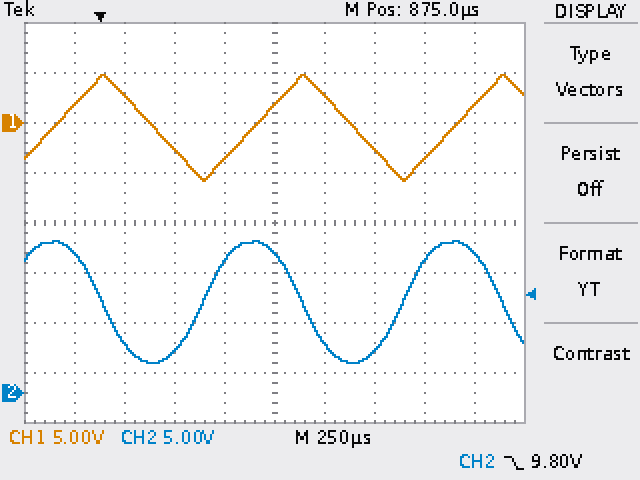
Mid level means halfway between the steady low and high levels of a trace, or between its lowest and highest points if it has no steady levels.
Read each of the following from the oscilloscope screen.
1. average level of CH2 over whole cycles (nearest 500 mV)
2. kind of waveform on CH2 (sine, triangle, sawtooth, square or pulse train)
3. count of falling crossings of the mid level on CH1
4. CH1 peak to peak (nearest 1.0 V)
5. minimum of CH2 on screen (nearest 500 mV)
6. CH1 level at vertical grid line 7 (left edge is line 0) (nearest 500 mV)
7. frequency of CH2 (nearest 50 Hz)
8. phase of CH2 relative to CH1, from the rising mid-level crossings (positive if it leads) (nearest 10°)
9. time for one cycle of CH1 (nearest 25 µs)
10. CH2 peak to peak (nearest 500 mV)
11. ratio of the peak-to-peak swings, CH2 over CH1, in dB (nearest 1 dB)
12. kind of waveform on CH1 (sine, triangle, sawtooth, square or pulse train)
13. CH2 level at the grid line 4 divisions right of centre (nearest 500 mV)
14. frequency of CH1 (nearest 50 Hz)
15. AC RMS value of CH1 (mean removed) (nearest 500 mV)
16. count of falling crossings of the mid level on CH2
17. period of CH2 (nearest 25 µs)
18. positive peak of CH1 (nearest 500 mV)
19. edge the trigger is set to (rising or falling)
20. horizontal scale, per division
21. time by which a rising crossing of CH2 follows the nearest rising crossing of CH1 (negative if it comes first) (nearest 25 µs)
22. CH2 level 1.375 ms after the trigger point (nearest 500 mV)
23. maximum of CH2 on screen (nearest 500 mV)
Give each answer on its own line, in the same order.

9.0 V
sine
2
11.0 V
3.0 V
-2.5 V
1.00 kHz
+90°
1.000 ms
12.0 V
1 dB
triangle
14.0 V
1.00 kHz
3.0 V
3
1.000 ms
5.0 V
falling
250 µs
-250 µs
4.0 V
15.0 V
